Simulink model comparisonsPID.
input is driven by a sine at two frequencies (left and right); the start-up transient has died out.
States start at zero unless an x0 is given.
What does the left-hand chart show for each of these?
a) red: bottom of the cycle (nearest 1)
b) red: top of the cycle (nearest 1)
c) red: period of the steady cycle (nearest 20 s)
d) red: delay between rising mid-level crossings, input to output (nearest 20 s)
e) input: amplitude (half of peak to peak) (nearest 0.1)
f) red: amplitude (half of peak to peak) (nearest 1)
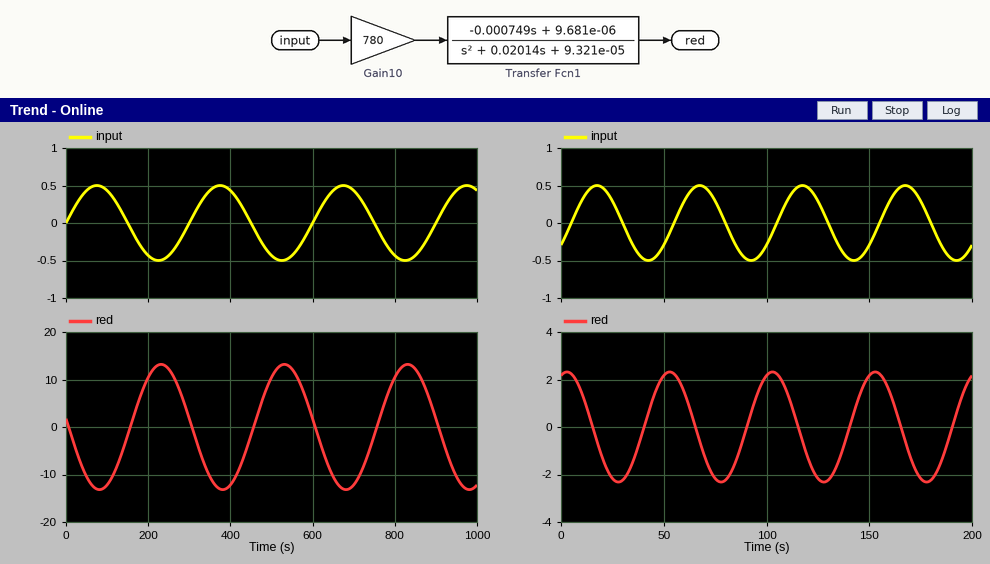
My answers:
-13
13
300 s
160 s
0.5
13
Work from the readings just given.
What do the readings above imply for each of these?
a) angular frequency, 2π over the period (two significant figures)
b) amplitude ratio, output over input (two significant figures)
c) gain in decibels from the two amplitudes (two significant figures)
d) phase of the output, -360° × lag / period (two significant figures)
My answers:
0.021 rad/s
26
28 dB
-190°
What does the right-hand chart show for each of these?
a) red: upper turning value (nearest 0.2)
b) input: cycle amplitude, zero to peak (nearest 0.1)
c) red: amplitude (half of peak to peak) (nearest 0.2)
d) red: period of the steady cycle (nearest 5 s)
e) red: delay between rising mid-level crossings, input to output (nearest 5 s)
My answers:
2.4
0.5
2.4
50 s
35 s
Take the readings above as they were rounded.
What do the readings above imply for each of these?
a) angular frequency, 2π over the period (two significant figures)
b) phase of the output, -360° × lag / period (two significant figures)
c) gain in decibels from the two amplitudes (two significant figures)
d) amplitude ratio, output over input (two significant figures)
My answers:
0.13 rad/s
-250°
14 dB
4.8
